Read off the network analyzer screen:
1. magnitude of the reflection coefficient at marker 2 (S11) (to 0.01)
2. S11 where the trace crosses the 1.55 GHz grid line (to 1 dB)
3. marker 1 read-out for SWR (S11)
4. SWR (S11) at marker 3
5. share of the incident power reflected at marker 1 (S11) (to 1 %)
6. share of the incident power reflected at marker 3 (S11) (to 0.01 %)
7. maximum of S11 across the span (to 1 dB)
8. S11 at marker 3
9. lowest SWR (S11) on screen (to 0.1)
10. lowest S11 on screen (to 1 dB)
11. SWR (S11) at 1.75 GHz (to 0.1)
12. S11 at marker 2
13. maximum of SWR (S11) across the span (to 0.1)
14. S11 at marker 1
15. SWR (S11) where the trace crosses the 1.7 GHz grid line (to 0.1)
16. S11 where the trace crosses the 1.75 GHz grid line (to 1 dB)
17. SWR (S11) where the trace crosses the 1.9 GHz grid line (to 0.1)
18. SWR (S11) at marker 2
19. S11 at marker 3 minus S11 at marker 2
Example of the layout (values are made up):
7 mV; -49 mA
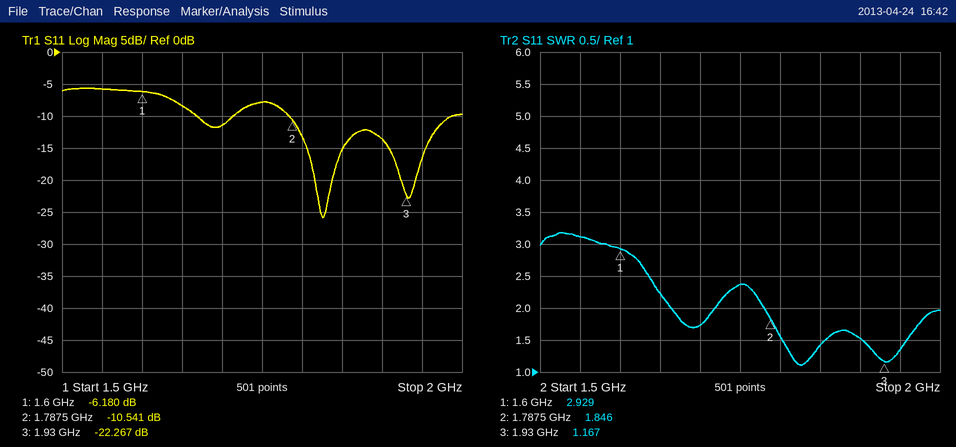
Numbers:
0.30; -6 dB; 2.929; 1.167; 24 %; 0.59 %; -6 dB; -22.267 dB; 1.1; -26 dB; 2.4; -10.541 dB; 3.2; -6.180 dB; 1.7; -8 dB; 1.5; 1.846; -11.726 dB
